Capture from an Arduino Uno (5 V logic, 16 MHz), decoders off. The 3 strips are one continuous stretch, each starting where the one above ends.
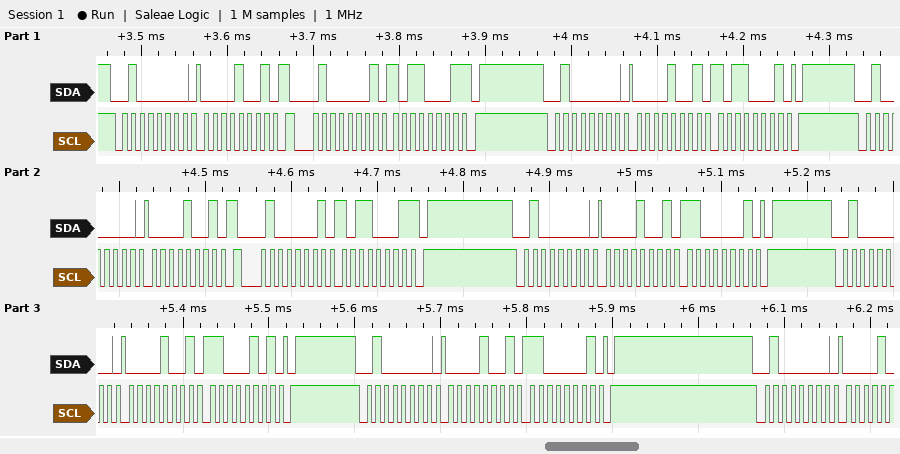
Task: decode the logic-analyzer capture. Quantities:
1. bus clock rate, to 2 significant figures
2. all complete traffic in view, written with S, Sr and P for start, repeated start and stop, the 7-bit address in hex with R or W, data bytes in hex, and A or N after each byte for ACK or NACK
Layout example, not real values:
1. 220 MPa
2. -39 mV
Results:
1. 100 kHz
2. S 20W A 09 A Sr 20R A B1 N P S 20W A 09 A B1 A P S 20W A 09 A Sr 20R A B1 N P S 20W A 09 A C1 A P S 20W A 09 A C5 A P S 20W A 09 A C1 A P S 20W A
